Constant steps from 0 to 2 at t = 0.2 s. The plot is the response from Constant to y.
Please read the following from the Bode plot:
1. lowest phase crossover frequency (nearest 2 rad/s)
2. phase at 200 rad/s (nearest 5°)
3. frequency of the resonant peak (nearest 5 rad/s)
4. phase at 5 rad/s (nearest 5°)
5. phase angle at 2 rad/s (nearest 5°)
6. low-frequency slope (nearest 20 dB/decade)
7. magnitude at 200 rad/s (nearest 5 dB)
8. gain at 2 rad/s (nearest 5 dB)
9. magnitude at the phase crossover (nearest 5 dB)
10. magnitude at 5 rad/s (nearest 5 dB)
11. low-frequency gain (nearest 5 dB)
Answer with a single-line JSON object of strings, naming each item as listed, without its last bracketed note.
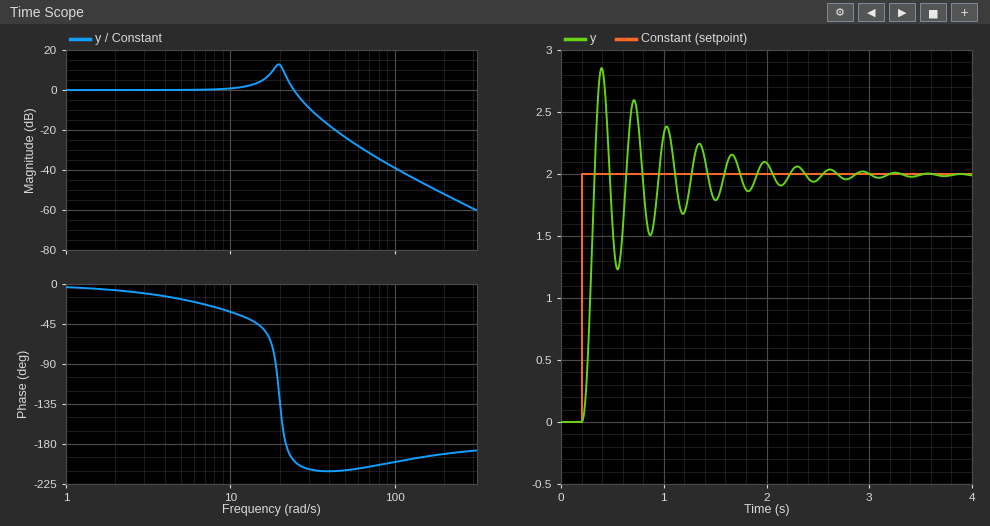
{"lowest phase crossover frequency": "22 rad/s", "phase at 200 rad/s": "-190°", "frequency of the resonant peak": "20 rad/s", "phase at 5 rad/s": "-15°", "phase angle at 2 rad/s": "-5°", "low-frequency slope": "0 dB/decade", "magnitude at 200 rad/s": "-50 dB", "gain at 2 rad/s": "0 dB", "magnitude at the phase crossover": "5 dB", "magnitude at 5 rad/s": "0 dB", "low-frequency gain": "0 dB"}
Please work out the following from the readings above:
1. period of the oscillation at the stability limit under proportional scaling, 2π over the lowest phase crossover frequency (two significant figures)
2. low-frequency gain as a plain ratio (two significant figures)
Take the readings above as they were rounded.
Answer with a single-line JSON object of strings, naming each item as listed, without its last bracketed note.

{"period of the oscillation at the stability limit under proportional scaling, 2π over the lowest phase crossover frequency": "0.29 s", "low-frequency gain as a plain ratio": "1.0"}
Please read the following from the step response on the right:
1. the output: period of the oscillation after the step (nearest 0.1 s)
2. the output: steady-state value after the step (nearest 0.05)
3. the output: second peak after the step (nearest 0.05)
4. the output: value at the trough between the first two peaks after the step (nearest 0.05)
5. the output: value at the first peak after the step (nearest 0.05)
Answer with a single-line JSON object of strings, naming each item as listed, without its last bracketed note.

{"the output: period of the oscillation after the step": "0.3 s", "the output: steady-state value after the step": "2.00", "the output: second peak after the step": "2.60", "the output: value at the trough between the first two peaks after the step": "1.25", "the output: value at the first peak after the step": "2.85"}
